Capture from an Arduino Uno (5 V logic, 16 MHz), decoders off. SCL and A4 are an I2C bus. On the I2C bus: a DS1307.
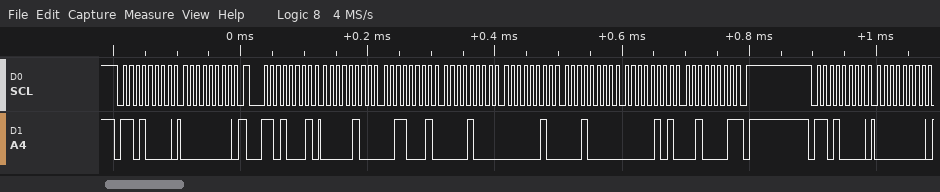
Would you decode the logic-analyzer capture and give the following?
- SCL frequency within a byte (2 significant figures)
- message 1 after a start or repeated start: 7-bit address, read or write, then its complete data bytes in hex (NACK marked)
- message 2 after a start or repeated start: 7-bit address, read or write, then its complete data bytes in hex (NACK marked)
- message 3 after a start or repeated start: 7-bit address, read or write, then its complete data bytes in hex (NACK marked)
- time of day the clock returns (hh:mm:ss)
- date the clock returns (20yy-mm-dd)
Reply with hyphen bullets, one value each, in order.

- 100 kHz
- 0x68 write: 00
- 0x68 read: 04 31 08 02 10 05 21 NACK
- 0x68 write: 00
- 08:31:04
- 2021-05-10
